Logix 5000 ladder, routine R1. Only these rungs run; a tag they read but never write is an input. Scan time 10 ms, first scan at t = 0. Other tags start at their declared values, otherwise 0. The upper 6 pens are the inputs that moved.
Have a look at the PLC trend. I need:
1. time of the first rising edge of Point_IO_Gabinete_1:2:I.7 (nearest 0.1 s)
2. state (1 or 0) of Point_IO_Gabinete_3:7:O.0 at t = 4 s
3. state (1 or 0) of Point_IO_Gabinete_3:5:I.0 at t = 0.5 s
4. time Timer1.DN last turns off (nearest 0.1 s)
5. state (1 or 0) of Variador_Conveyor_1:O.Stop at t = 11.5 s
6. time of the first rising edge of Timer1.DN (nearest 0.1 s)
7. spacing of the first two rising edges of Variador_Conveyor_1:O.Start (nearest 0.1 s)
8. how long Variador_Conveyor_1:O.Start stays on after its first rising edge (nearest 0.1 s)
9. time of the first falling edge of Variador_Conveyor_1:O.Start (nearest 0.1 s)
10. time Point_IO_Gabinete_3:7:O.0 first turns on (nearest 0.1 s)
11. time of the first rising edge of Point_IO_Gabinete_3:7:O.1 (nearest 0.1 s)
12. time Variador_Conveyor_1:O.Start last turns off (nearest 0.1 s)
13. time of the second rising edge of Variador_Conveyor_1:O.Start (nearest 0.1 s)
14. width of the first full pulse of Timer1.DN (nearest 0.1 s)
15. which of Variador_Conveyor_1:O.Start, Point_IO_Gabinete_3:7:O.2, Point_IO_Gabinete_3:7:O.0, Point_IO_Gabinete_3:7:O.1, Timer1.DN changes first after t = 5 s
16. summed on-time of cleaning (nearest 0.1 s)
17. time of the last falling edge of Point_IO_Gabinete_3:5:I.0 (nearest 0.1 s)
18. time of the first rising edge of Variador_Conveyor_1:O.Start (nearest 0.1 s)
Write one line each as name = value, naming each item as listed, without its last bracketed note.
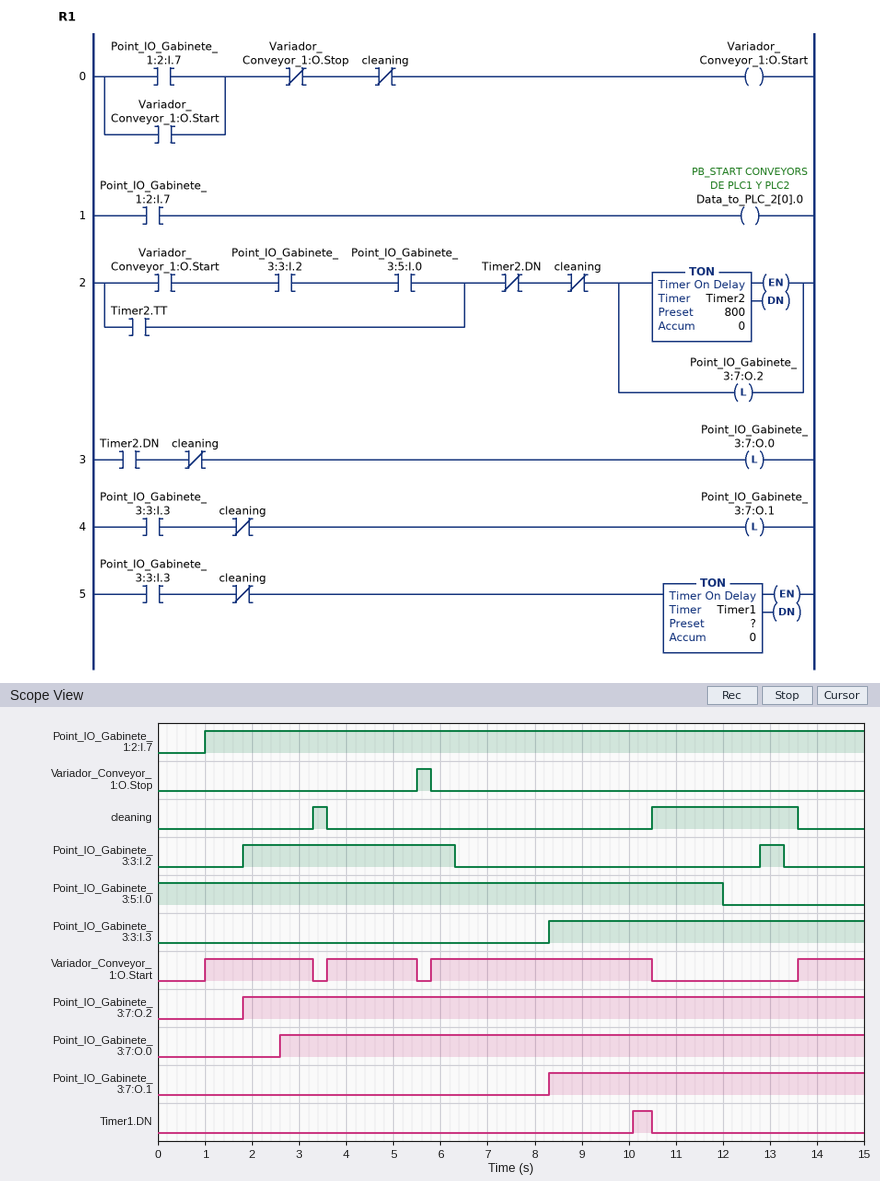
time of the first rising edge of Point_IO_Gabinete_1:2:I.7 = 1.0 s
state (1 or 0) of Point_IO_Gabinete_3:7:O.0 at t = 4 s = 1
state (1 or 0) of Point_IO_Gabinete_3:5:I.0 at t = 0.5 s = 1
time Timer1.DN last turns off = 10.5 s
state (1 or 0) of Variador_Conveyor_1:O.Stop at t = 11.5 s = 0
time of the first rising edge of Timer1.DN = 10.1 s
spacing of the first two rising edges of Variador_Conveyor_1:O.Start = 2.6 s
how long Variador_Conveyor_1:O.Start stays on after its first rising edge = 2.3 s
time of the first falling edge of Variador_Conveyor_1:O.Start = 3.3 s
time Point_IO_Gabinete_3:7:O.0 first turns on = 2.6 s
time of the first rising edge of Point_IO_Gabinete_3:7:O.1 = 8.3 s
time Variador_Conveyor_1:O.Start last turns off = 10.5 s
time of the second rising edge of Variador_Conveyor_1:O.Start = 3.6 s
width of the first full pulse of Timer1.DN = 0.4 s
which of Variador_Conveyor_1:O.Start, Point_IO_Gabinete_3:7:O.2, Point_IO_Gabinete_3:7:O.0, Point_IO_Gabinete_3:7:O.1, Timer1.DN changes first after t = 5 s = Variador_Conveyor_1:O.Start
summed on-time of cleaning = 3.4 s
time of the last falling edge of Point_IO_Gabinete_3:5:I.0 = 12.0 s
time of the first rising edge of Variador_Conveyor_1:O.Start = 1.0 s
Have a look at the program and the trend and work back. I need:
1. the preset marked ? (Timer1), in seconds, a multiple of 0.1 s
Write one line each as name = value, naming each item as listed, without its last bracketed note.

the preset marked ? (Timer1), in seconds, a multiple of 0.1 s = 1.8 s
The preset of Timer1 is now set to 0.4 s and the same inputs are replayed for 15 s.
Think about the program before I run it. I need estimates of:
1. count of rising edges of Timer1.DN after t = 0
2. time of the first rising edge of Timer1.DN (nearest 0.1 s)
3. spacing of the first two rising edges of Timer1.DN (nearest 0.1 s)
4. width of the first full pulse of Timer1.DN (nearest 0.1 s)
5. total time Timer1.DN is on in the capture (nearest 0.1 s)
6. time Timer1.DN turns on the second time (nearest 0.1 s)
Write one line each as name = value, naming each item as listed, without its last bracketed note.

count of rising edges of Timer1.DN after t = 0 = 2
time of the first rising edge of Timer1.DN = 8.7 s
spacing of the first two rising edges of Timer1.DN = 5.3 s
width of the first full pulse of Timer1.DN = 1.8 s
total time Timer1.DN is on in the capture = 2.8 s
time Timer1.DN turns on the second time = 14.0 s
